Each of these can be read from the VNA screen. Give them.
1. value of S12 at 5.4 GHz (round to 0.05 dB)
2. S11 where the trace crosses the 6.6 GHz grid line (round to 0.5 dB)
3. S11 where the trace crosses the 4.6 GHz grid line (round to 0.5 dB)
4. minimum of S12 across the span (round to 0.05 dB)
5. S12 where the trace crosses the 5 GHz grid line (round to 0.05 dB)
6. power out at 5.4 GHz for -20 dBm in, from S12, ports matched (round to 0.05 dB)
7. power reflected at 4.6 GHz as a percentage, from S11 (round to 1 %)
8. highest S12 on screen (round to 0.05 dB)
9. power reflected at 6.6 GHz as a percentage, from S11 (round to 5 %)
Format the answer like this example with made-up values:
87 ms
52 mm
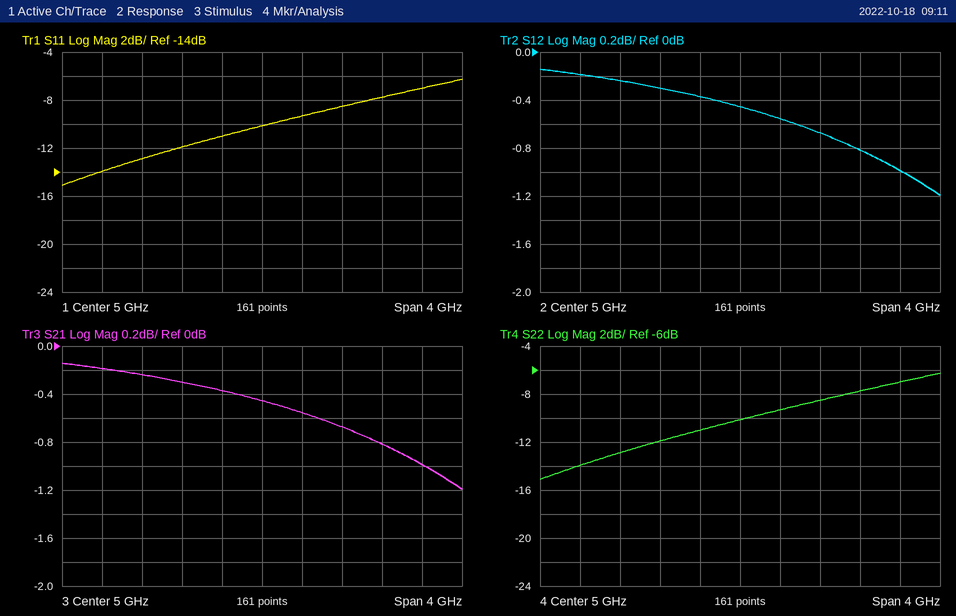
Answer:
-0.55 dB
-7.0 dB
-11.0 dB
-1.20 dB
-0.45 dB
-20.55 dBm
8 %
-0.15 dB
20 %
